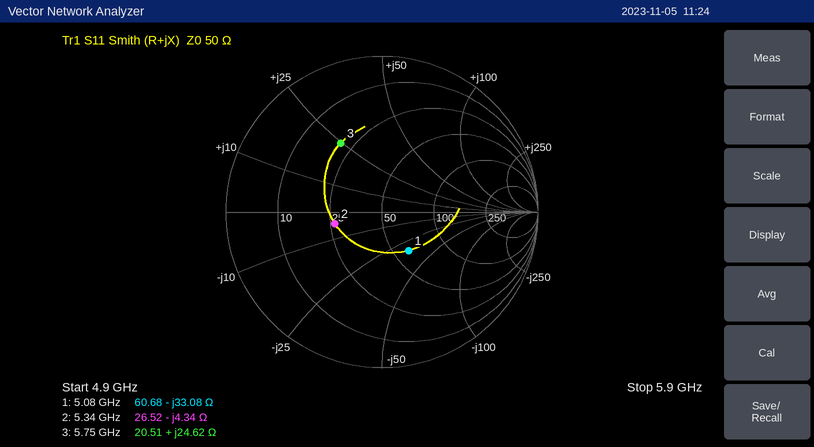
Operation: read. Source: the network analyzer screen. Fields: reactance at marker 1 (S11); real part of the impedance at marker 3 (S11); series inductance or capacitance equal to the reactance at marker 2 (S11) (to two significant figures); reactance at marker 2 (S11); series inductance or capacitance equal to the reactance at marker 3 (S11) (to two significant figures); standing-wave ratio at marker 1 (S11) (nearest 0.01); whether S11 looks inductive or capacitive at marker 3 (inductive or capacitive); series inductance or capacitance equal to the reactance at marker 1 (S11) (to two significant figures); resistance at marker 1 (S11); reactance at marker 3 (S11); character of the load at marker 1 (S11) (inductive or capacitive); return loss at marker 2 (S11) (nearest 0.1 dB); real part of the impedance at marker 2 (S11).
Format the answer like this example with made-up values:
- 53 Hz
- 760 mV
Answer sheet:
- -33.08 Ω
- 20.51 Ω
- 6.9 pF
- -4.34 Ω
- 680 pH
- 1.86
- inductive
- 950 fF
- 60.68 Ω
- +24.62 Ω
- capacitive
- 10.1 dB
- 26.52 Ω
